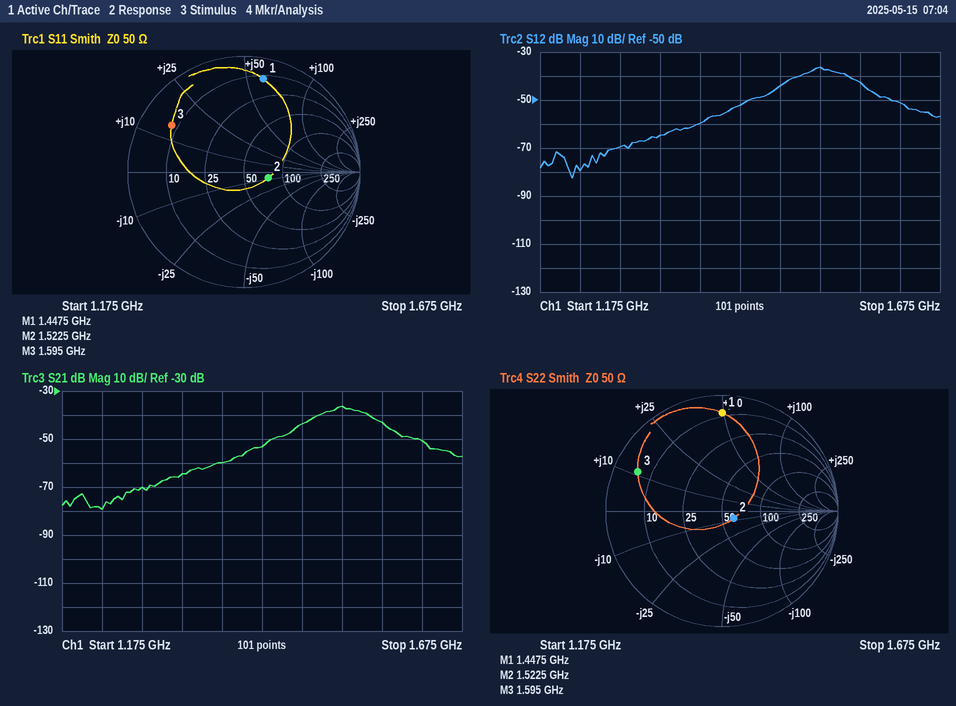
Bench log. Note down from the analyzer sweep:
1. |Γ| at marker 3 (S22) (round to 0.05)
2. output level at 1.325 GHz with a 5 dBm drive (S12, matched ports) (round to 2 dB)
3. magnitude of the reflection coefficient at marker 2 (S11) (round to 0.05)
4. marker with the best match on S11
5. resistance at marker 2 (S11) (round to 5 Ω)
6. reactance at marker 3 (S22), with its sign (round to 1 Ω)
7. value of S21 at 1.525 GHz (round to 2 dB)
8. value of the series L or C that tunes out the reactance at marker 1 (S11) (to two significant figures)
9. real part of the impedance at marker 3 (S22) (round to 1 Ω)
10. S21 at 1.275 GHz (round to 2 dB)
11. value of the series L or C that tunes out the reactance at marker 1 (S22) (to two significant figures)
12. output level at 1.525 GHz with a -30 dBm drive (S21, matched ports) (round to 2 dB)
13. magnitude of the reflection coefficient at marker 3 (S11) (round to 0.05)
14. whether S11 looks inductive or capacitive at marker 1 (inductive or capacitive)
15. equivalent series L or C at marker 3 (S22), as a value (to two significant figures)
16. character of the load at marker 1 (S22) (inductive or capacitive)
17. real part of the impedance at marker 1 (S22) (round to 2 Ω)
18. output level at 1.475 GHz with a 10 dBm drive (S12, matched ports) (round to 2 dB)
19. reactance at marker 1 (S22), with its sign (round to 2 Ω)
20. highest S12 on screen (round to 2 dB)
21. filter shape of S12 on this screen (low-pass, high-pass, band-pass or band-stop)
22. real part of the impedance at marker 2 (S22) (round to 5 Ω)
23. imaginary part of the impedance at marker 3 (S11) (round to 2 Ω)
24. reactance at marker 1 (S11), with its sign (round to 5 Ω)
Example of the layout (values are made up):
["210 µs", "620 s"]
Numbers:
["0.80", "-60 dBm", "0.20", "marker 2", "75 Ω", "+11 Ω", "-36 dB", "1.8 pF", "6 Ω", "-70 dB", "2.2 pF", "-66 dBm", "0.75", "inductive", "1.1 nH", "inductive", "8 Ω", "-34 dBm", "+50 Ω", "-36 dB", "band-pass", "60 Ω", "+14 Ω", "+60 Ω"]
